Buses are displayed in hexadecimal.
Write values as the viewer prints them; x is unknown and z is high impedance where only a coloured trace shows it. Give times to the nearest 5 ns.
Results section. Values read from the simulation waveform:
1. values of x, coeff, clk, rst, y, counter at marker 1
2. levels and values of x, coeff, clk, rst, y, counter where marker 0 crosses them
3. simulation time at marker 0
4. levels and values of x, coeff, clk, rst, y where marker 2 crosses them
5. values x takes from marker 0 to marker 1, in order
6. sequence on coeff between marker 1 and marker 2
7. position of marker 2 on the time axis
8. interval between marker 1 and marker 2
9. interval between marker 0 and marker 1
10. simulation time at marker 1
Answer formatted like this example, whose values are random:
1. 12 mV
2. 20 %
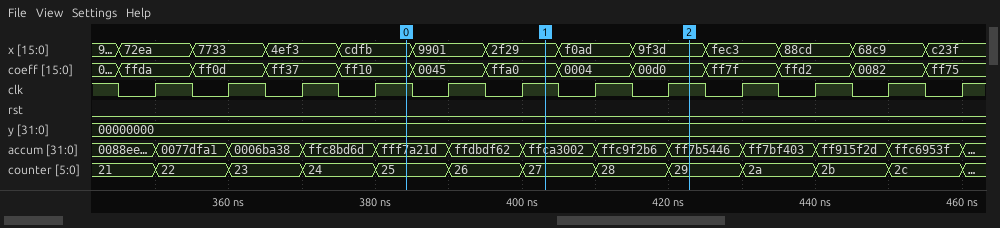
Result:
1. x=2f29, coeff=ffa0, clk=1, rst=0, y=00000000, counter=27
2. x=cdfb, coeff=ff10, clk=1, rst=0, y=00000000, counter=25
3. 385 ns
4. x=9f3d, coeff=00d0, clk=1, rst=0, y=00000000
5. cdfb, 9901, 2f29
6. ffa0, 0004, 00d0
7. 425 ns
8. 20 ns
9. 20 ns
10. 405 ns
